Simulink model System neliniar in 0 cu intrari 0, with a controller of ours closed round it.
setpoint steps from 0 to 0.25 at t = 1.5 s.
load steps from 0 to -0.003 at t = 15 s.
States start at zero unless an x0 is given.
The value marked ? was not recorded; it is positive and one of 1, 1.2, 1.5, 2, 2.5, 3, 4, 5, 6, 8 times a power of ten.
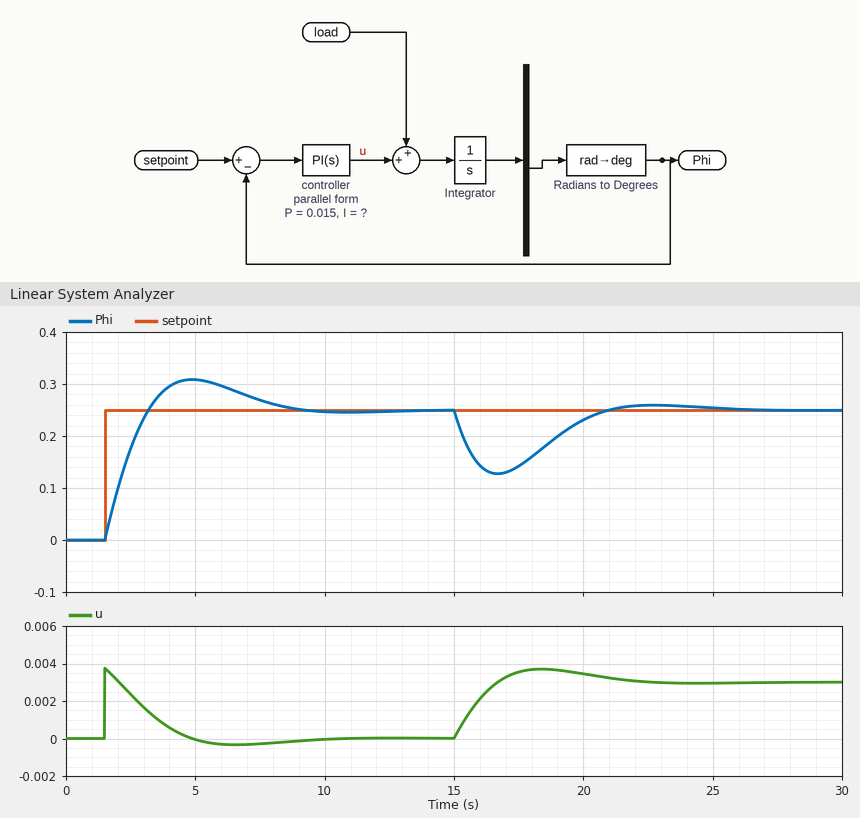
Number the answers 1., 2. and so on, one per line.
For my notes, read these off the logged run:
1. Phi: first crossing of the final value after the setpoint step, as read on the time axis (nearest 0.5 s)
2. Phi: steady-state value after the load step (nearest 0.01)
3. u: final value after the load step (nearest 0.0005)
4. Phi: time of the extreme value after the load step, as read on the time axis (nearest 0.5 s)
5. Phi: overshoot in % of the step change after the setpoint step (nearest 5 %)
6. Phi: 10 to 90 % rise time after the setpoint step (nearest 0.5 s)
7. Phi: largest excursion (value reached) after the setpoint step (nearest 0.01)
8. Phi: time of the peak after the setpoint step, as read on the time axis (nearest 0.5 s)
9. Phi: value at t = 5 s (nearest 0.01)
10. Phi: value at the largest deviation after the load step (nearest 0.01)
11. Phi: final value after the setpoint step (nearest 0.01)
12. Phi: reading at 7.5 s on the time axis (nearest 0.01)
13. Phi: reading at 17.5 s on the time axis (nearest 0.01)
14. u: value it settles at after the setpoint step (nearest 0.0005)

1. 3.0 s
2. 0.25
3. 0.0030
4. 16.5 s
5. 25 %
6. 1.5 s
7. 0.31
8. 5.0 s
9. 0.31
10. 0.13
11. 0.25
12. 0.27
13. 0.14
14. 0.0000
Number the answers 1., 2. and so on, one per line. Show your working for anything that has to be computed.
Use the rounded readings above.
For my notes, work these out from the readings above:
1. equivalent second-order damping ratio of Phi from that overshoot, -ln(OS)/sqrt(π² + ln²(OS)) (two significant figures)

1. ln(0.25) = -1.386; 1.386 / sqrt(9.870 + 1.922) = 0.40
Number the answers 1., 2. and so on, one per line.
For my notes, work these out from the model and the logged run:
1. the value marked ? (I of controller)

1. 0.008
